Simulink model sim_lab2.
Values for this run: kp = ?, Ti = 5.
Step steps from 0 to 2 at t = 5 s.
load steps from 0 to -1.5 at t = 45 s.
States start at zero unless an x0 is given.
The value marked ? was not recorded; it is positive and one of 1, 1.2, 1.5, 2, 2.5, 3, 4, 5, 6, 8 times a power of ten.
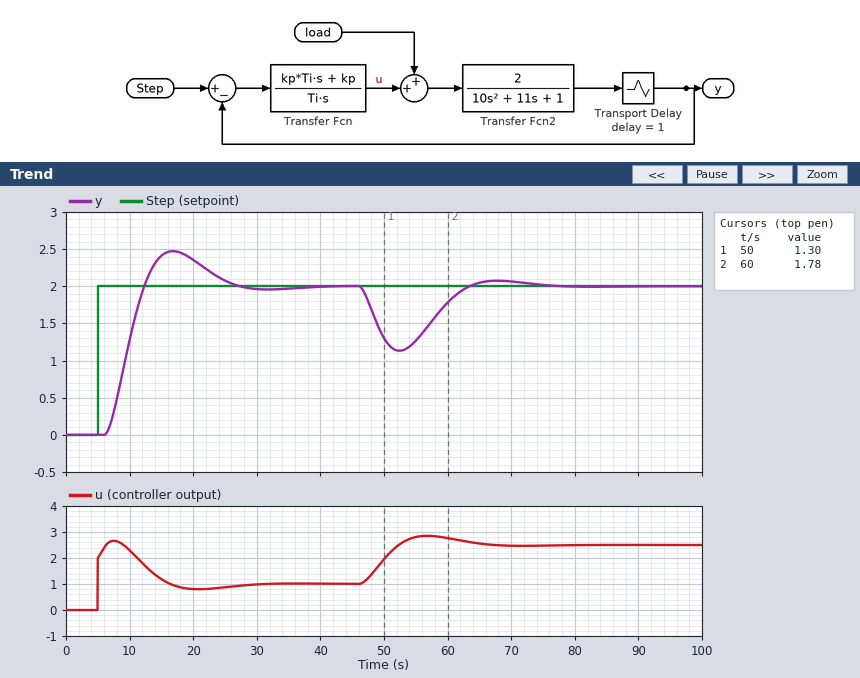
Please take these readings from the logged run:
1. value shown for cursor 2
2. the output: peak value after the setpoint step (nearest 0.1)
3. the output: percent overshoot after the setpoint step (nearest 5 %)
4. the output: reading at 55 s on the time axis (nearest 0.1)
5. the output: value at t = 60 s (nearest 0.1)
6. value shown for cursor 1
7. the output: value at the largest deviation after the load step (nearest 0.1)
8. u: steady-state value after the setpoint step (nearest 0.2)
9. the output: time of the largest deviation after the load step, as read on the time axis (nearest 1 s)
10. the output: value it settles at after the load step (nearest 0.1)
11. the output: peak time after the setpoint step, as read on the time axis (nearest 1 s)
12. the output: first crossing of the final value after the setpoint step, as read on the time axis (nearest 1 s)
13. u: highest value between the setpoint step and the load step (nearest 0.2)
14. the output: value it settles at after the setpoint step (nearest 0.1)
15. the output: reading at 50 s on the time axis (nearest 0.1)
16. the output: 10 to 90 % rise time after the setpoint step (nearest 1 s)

1.78
2.5
25 %
1.3
1.8
1.30
1.1
1.0
52 s
2.0
17 s
12 s
2.6
2.0
1.3
4 s
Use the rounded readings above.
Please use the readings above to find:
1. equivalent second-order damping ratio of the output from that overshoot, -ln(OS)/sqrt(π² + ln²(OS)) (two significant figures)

0.40
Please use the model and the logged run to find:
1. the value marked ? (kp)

1
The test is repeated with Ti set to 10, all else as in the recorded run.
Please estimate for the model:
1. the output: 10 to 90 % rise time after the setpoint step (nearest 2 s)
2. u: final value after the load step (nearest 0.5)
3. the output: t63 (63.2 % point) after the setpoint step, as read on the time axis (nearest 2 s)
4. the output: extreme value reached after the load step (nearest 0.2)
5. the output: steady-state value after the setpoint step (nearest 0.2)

6 s
2.5
10 s
1.0
2.0
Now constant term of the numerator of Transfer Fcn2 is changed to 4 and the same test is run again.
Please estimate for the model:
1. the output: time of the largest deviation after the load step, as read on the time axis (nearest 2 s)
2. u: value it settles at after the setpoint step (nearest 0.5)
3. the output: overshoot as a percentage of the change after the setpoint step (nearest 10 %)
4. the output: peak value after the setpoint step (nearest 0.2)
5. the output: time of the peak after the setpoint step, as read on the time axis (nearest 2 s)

50 s
0.5
50 %
3.0
12 s
